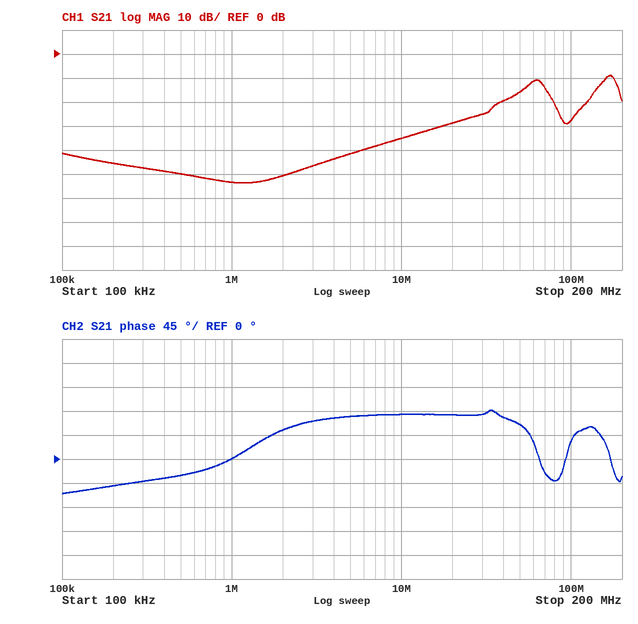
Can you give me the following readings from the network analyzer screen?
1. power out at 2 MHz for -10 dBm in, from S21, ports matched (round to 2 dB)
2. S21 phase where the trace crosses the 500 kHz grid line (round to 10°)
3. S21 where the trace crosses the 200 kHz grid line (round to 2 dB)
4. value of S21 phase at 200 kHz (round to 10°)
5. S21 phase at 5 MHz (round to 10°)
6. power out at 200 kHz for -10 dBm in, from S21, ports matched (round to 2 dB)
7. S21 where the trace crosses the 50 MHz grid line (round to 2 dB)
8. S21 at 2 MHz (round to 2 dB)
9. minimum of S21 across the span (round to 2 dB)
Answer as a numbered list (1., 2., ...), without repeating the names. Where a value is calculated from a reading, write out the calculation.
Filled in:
1. -10 dBm + (-50 dB) = -60 dBm
2. -30°
3. -46 dB
4. -50°
5. 80°
6. -10 dBm + (-46 dB) = -56 dBm
7. -16 dB
8. -50 dB
9. -54 dB
